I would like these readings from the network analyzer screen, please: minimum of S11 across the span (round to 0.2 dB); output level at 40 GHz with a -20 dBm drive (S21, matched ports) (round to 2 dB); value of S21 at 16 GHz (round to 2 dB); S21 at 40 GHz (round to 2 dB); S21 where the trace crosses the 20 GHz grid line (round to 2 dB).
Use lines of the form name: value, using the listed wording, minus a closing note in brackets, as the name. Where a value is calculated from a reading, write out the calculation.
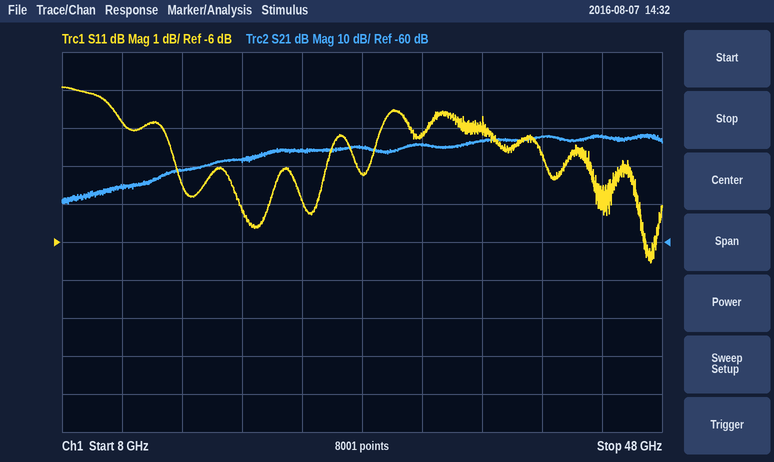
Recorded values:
minimum of S11 across the span: -6.6 dB
output level at 40 GHz with a -20 dBm drive (S21, matched ports): -20 dBm + (-32 dB) = -52 dBm
value of S21 at 16 GHz: -42 dB
S21 at 40 GHz: -32 dB
S21 where the trace crosses the 20 GHz grid line: -38 dB
